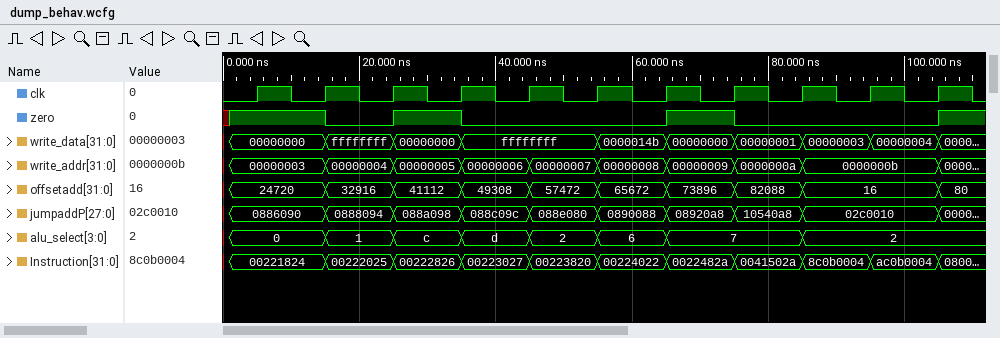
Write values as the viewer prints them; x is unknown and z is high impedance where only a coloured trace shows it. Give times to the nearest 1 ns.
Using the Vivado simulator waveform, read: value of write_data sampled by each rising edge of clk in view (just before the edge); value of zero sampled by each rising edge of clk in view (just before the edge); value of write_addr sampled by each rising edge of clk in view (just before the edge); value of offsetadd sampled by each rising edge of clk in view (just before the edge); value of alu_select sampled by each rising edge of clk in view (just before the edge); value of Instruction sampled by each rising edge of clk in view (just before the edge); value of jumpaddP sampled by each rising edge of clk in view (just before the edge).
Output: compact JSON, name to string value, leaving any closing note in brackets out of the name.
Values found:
{"value of write_data sampled by each rising edge of clk in view": "00000000, 00000000, ffffffff, 00000000, ffffffff, ffffffff, 0000014b, 00000000, 00000001, 00000003, 00000004", "value of zero sampled by each rising edge of clk in view": "1 1 0 1 0 0 0 1 0 0 0", "value of write_addr sampled by each rising edge of clk in view": "00000003, 00000003, 00000004, 00000005, 00000006, 00000007, 00000008, 00000009, 0000000a, 0000000b, 0000000b", "value of offsetadd sampled by each rising edge of clk in view": "24720, 24720, 32916, 41112, 49308, 57472, 65672, 73896, 82088, 16, 16", "value of alu_select sampled by each rising edge of clk in view": "0, 0, 1, c, d, 2, 6, 7, 7, 2, 2", "value of Instruction sampled by each rising edge of clk in view": "00221824, 00221824, 00222025, 00222826, 00223027, 00223820, 00224022, 0022482a, 0041502a, 8c0b0004, ac0b0004", "value of jumpaddP sampled by each rising edge of clk in view": "0886090, 0886090, 0888094, 088a098, 088c09c, 088e080, 0890088, 08920a8, 10540a8, 02c0010, 02c0010"}
